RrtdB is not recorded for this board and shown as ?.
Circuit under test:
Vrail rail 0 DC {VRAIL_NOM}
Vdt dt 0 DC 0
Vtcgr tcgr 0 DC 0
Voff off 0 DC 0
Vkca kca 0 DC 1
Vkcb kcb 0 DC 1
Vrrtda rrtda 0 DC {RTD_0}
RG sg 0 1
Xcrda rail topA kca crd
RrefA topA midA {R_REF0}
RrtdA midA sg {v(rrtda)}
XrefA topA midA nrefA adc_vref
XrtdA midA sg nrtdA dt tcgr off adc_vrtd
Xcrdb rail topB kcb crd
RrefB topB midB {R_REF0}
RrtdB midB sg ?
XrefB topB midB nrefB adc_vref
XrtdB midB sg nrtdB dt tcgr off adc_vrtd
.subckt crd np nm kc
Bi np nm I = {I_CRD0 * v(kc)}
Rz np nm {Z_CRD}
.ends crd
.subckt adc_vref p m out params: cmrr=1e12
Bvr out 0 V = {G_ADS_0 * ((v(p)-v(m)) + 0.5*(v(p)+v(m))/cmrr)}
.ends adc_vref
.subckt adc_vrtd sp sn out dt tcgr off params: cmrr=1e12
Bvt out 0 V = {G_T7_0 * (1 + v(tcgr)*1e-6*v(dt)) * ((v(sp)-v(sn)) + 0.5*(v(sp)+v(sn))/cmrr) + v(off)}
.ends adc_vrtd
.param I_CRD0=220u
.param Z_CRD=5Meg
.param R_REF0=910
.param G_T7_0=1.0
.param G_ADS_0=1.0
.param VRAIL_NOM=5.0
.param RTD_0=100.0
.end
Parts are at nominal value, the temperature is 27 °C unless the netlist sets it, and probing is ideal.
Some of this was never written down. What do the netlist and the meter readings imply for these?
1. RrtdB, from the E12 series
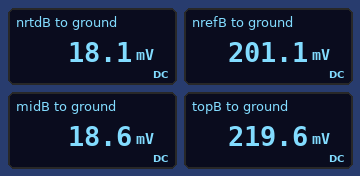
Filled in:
82 Ω
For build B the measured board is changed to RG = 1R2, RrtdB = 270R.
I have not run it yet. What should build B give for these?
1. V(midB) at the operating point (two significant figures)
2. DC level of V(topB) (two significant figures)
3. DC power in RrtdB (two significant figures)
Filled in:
60 mV
260 mV
13 µW
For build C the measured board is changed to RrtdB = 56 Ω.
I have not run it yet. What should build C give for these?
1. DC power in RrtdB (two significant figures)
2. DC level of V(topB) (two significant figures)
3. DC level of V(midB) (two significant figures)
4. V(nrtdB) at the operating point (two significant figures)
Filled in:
2.7 µW
210 mV
13 mV
12 mV
